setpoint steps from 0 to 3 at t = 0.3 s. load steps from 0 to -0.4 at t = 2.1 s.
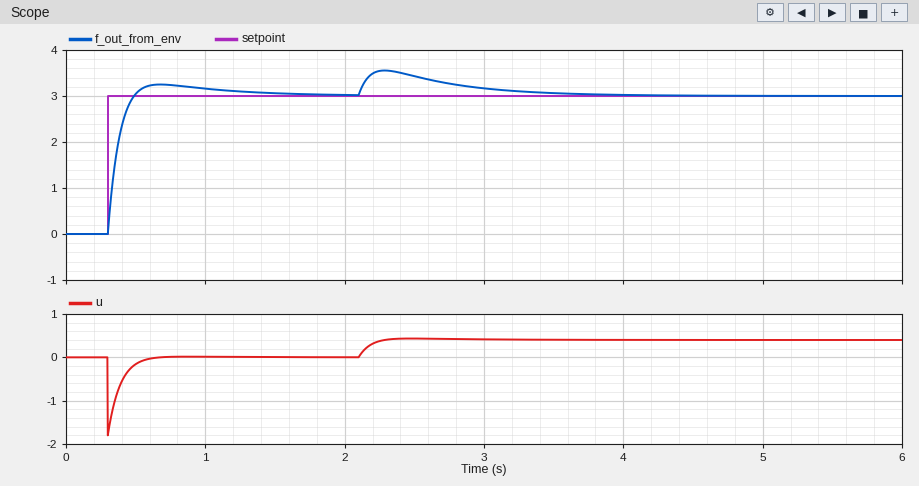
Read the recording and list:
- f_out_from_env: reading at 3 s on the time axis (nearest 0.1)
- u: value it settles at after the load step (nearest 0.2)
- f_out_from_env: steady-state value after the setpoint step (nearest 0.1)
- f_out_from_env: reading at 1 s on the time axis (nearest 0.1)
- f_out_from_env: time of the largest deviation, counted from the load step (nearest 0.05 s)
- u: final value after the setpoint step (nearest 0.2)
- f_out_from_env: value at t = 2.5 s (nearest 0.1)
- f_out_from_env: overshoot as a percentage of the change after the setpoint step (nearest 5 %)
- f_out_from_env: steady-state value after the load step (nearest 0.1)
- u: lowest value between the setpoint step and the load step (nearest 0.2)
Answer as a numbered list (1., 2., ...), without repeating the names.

1. 3.2
2. 0.4
3. 3.0
4. 3.2
5. 0.20 s
6. 0.0
7. 3.4
8. 10 %
9. 3.0
10. -1.8
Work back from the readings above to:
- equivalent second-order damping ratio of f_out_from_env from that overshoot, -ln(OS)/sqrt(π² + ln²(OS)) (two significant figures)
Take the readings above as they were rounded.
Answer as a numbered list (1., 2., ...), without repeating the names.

1. 0.59
